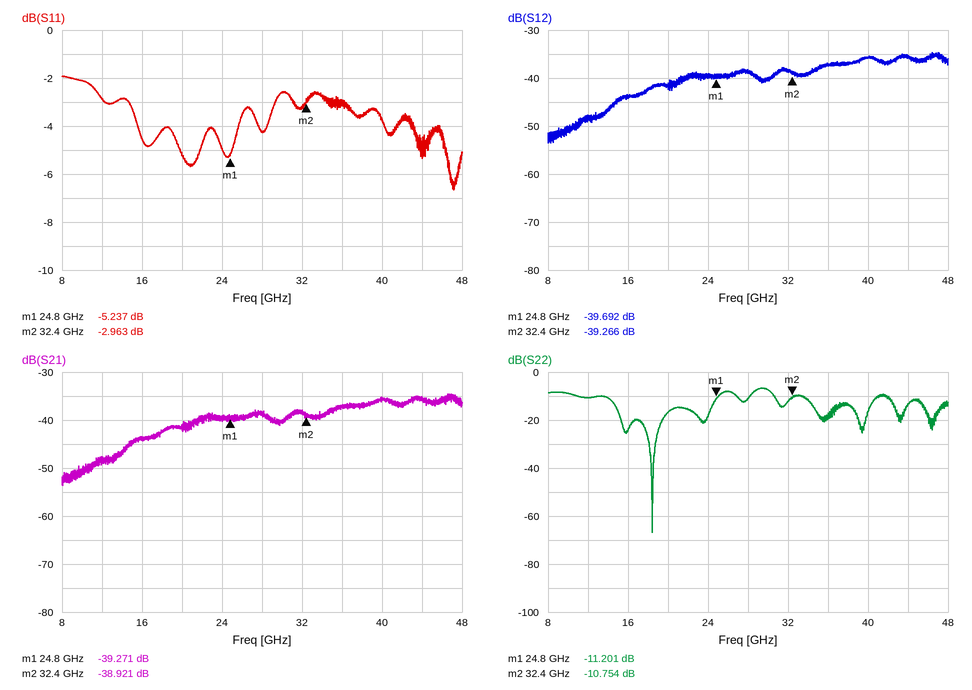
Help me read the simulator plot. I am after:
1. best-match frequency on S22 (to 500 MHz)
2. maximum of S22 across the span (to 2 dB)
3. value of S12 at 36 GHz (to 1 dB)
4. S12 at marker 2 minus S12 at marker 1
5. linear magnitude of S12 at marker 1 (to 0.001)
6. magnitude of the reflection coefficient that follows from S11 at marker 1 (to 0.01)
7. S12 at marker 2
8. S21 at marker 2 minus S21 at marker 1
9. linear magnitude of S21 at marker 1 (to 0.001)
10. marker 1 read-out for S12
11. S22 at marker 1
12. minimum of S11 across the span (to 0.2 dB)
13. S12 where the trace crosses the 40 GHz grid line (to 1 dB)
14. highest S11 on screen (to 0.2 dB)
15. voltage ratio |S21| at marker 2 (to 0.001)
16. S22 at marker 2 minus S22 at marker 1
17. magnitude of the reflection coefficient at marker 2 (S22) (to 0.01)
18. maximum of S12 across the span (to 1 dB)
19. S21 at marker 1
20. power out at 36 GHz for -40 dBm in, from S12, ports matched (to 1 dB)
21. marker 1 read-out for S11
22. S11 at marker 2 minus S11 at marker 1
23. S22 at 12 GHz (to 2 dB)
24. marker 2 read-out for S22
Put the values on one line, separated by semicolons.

18.5 GHz; -6 dB; -37 dB; 0.426 dB; 0.010; 0.55; -39.266 dB; 0.350 dB; 0.011; -39.692 dB; -11.201 dB; -6.6 dB; -36 dB; -2.0 dB; 0.011; 0.447 dB; 0.29; -35 dB; -39.271 dB; -77 dBm; -5.237 dB; 2.274 dB; -10 dB; -10.754 dB
